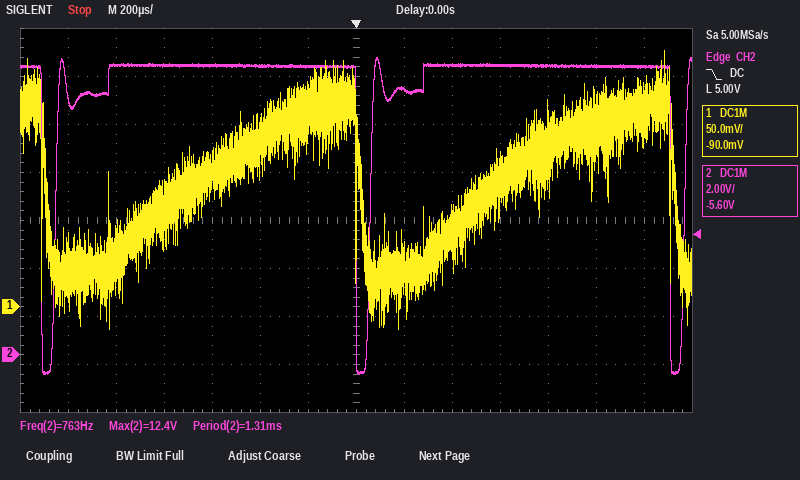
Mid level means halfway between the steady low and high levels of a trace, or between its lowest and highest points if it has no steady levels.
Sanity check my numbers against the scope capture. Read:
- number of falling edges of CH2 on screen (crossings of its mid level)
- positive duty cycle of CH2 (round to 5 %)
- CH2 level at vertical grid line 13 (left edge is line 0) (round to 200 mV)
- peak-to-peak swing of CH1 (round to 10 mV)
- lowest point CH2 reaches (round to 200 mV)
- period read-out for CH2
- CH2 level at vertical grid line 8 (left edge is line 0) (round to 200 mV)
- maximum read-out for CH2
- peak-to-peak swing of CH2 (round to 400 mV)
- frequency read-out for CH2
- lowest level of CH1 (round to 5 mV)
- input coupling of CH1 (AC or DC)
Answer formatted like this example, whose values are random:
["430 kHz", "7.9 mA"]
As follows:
["3", "95 %", "12.0 V", "290 mV", "-800 mV", "1.31 ms", "11.0 V", "12.4 V", "13.2 V", "763 Hz", "-25 mV", "DC"]
